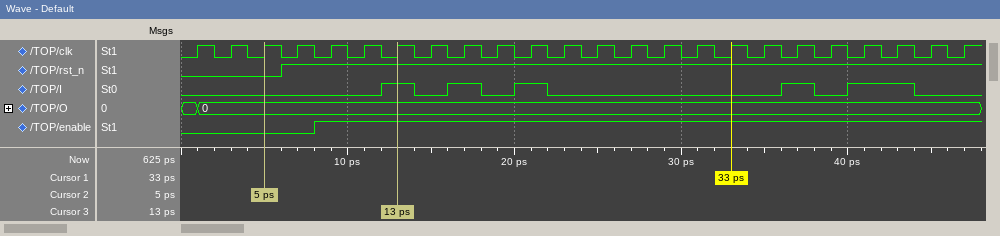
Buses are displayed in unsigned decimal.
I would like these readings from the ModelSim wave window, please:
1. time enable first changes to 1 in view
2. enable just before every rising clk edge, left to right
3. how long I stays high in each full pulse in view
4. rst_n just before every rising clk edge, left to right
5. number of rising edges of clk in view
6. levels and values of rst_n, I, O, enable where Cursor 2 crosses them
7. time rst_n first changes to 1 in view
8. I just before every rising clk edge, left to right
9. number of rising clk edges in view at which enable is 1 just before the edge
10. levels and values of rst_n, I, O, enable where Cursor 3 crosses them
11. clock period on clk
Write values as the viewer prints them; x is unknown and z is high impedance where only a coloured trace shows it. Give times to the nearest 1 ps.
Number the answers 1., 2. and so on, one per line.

1. 8 ps
2. 0 0 0 0 1 1 1 1 1 1 1 1 1 1 1 1 1 1 1 1 1 1 1 1
3. 2 ps, 2 ps, 2 ps, 2 ps, 4 ps
4. 0 0 0 1 1 1 1 1 1 1 1 1 1 1 1 1 1 1 1 1 1 1 1 1
5. 24
6. rst_n=0, I=0, O=0, enable=0
7. 6 ps
8. 0 0 0 0 0 0 1 0 1 0 1 0 0 0 0 0 0 0 1 0 1 1 0 0
9. 20
10. rst_n=1, I=1, O=0, enable=1
11. 2 ps
